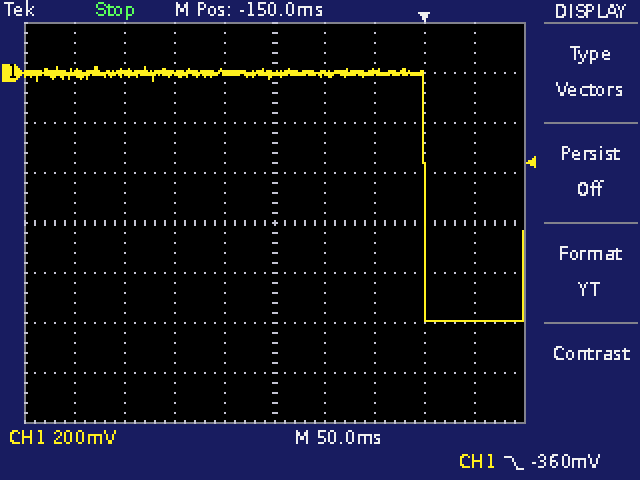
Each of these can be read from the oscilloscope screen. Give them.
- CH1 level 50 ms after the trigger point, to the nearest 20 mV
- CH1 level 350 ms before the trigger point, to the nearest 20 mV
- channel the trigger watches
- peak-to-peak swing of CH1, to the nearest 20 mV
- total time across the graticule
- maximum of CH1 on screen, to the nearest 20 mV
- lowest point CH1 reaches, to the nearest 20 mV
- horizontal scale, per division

-1.00 V
0 mV
CH1
1.02 V
500 ms
20 mV
-1.00 V
50 ms
